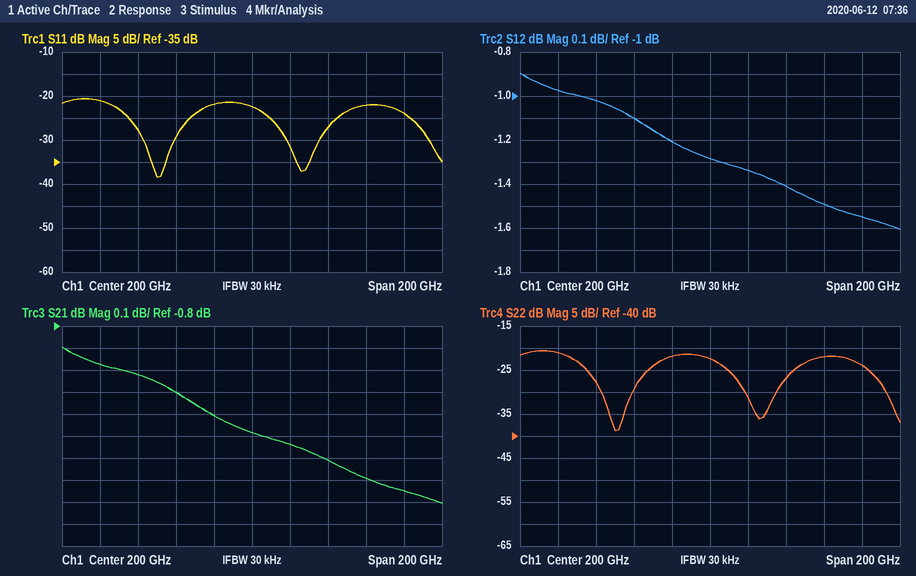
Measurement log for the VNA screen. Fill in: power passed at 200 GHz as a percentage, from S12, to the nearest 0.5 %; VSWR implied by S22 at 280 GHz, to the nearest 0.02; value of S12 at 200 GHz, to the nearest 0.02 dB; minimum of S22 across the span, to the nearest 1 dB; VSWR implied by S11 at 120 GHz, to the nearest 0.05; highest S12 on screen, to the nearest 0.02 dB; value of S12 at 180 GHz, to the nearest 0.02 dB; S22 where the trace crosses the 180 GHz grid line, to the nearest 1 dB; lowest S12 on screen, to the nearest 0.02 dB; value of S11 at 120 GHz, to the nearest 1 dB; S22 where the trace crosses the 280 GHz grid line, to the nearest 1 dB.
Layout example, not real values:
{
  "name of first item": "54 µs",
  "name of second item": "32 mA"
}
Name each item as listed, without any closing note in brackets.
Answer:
{
  "power passed at 200 GHz as a percentage, from S12, to the nearest 0.5 %": "74.5 %",
  "VSWR implied by S22 at 280 GHz, to the nearest 0.02": "1.14",
  "value of S12 at 200 GHz, to the nearest 0.02 dB": "-1.28 dB",
  "minimum of S22 across the span, to the nearest 1 dB": "-39 dB",
  "VSWR implied by S11 at 120 GHz, to the nearest 0.05": "1.20",
  "highest S12 on screen, to the nearest 0.02 dB": "-0.90 dB",
  "value of S12 at 180 GHz, to the nearest 0.02 dB": "-1.20 dB",
  "S22 where the trace crosses the 180 GHz grid line, to the nearest 1 dB": "-22 dB",
  "lowest S12 on screen, to the nearest 0.02 dB": "-1.60 dB",
  "value of S11 at 120 GHz, to the nearest 1 dB": "-21 dB",
  "S22 where the trace crosses the 280 GHz grid line, to the nearest 1 dB": "-24 dB"
}
